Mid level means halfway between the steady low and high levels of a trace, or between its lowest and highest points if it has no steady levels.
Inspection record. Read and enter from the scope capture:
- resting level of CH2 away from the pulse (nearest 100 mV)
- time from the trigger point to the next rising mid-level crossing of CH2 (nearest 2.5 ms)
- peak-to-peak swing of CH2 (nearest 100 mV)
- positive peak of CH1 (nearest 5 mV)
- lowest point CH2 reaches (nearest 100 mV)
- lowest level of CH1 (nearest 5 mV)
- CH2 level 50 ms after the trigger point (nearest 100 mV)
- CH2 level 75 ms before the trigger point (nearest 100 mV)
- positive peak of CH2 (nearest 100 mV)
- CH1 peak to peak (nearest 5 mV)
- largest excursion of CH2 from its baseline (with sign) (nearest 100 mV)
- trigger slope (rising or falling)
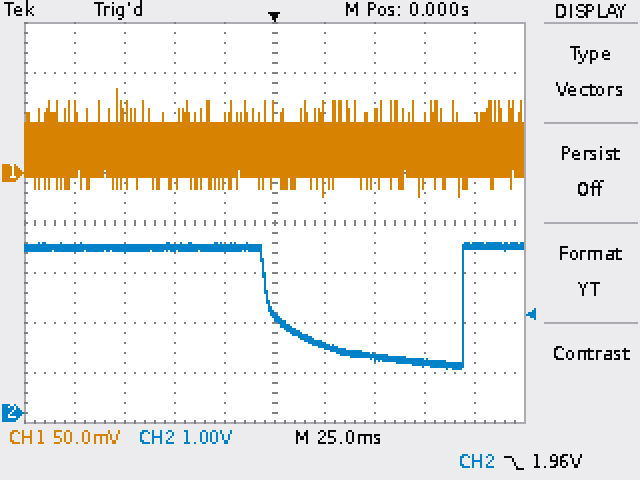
3.3 V
95.0 ms
2.5 V
85 mV
900 mV
-25 mV
1.1 V
3.3 V
3.4 V
110 mV
-2.4 V
falling
